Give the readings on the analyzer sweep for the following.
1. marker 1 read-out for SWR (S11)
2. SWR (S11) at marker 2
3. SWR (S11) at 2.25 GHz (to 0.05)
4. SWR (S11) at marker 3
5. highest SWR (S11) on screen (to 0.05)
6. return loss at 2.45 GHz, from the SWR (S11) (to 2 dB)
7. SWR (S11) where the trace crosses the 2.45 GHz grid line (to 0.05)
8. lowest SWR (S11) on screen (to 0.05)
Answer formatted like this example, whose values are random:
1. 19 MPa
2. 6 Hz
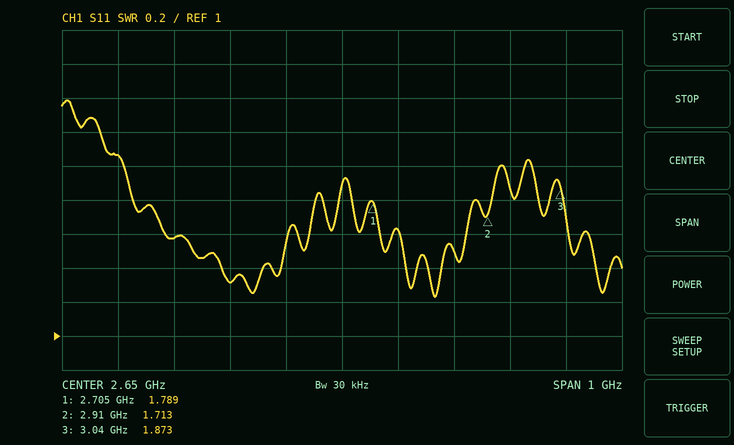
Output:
1. 1.789
2. 1.713
3. 2.05
4. 1.873
5. 2.40
6. 18 dB
7. 1.30
8. 1.25
